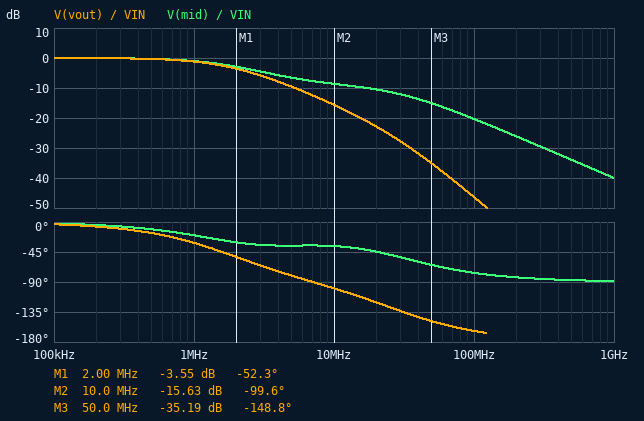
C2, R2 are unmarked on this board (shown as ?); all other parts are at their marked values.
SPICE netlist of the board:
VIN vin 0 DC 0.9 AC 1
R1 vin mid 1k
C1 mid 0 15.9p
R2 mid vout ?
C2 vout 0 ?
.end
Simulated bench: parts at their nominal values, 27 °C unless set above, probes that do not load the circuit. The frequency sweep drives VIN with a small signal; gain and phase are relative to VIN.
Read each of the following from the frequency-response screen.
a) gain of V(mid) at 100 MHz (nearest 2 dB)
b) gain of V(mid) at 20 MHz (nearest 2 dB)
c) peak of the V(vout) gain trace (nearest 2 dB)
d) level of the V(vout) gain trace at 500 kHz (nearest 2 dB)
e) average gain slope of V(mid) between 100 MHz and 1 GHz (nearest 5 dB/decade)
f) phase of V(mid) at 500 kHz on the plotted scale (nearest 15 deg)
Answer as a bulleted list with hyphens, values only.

- -20 dB
- -10 dB
- 0 dB
- 0 dB
- -20 dB/decade
- -15 deg
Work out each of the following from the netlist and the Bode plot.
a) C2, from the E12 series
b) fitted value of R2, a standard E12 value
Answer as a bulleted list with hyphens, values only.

- 47 pF
- 680 Ω
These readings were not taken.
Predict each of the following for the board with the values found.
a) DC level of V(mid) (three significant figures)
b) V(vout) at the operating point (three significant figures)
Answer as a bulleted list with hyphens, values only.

- 900 mV
- 900 mV
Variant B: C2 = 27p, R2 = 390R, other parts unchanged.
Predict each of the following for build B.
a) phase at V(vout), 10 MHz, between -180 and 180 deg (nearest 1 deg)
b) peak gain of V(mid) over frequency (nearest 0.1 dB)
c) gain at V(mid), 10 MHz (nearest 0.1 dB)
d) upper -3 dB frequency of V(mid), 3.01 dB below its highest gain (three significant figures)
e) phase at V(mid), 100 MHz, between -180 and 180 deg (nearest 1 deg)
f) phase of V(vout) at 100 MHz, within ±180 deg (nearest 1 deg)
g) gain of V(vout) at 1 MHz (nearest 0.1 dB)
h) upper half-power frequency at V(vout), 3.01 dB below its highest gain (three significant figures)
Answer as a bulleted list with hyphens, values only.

- -84 deg
- 0 dB
- -9.0 dB
- 3.31 MHz
- -71 deg
- -153 deg
- -0.4 dB
- 3.16 MHz
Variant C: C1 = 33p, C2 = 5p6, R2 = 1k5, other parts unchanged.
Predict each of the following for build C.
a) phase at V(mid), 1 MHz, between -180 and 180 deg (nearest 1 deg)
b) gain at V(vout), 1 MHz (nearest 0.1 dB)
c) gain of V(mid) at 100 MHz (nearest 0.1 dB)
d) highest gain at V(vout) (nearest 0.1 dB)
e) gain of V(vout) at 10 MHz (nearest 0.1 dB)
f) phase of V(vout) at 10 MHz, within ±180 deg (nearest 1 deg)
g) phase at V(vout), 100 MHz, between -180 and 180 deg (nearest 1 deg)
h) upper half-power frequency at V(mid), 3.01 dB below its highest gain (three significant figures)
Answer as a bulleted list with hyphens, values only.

- -14 deg
- -0.3 dB
- -26.4 dB
- 0 dB
- -9.4 dB
- -92 deg
- -165 deg
- 4.03 MHz
